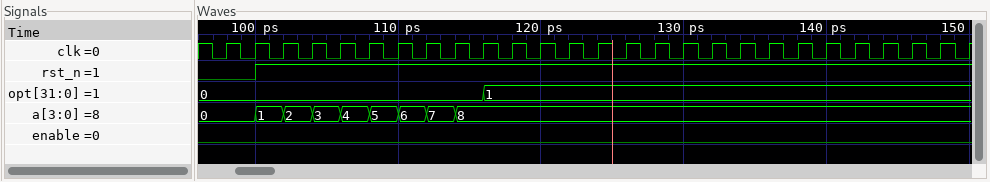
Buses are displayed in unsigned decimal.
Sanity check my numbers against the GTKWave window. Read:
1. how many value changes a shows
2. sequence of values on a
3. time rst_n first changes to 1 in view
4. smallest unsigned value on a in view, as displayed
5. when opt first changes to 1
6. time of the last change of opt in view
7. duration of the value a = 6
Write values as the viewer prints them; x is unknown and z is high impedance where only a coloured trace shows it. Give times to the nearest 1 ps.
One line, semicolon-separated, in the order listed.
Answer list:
8; 0, 1, 2, 3, 4, 5, 6, 7, 8; 100 ps; 0; 116 ps; 116 ps; 2 ps
